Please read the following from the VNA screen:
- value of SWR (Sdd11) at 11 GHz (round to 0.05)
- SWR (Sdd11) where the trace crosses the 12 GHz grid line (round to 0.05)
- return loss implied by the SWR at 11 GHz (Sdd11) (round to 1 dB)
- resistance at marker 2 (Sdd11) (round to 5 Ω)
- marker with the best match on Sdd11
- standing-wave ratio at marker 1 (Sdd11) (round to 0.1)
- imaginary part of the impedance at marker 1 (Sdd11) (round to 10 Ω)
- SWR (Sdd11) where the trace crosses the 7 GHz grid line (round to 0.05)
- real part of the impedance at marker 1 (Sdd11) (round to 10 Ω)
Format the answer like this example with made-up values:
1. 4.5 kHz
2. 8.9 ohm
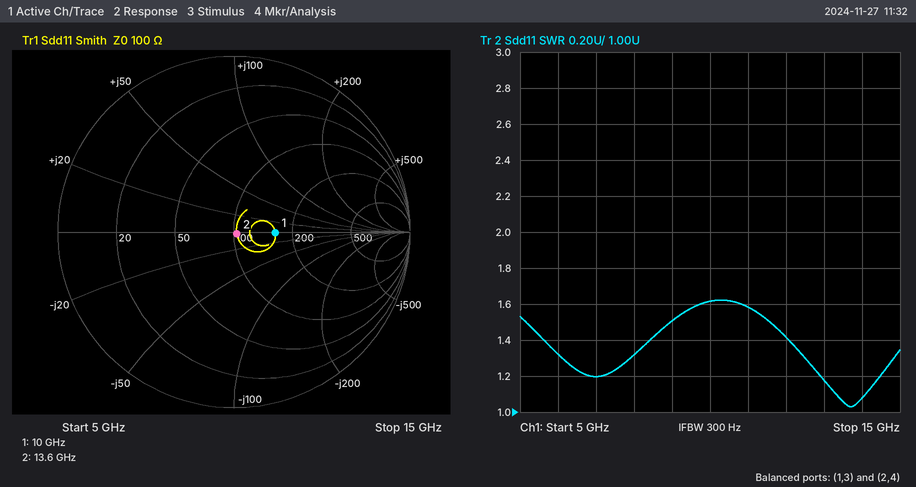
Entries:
1. 1.60
2. 1.40
3. 13 dB
4. 105 Ω
5. marker 2
6. 1.6
7. 0 Ω
8. 1.20
9. 160 Ω
